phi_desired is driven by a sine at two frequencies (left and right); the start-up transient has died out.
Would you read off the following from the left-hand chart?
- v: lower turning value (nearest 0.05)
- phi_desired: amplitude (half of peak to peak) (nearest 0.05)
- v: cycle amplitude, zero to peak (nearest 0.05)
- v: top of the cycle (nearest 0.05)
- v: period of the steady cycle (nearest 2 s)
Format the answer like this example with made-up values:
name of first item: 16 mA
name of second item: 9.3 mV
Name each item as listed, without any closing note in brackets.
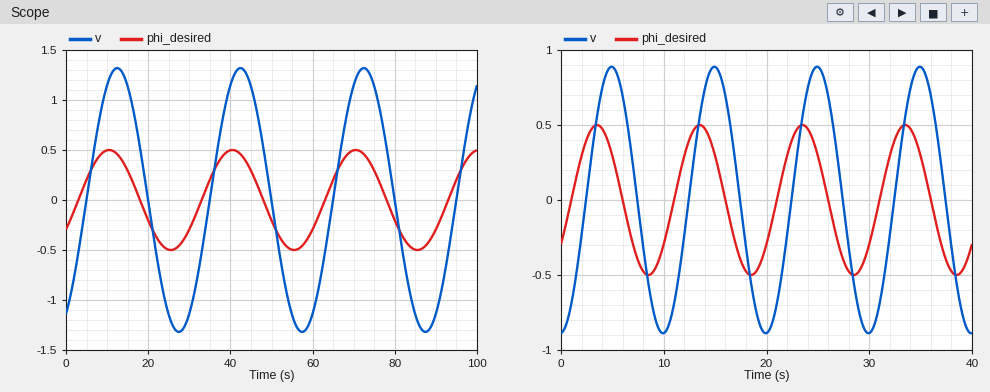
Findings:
v: lower turning value: -1.30
phi_desired: amplitude (half of peak to peak): 0.50
v: cycle amplitude, zero to peak: 1.30
v: top of the cycle: 1.30
v: period of the steady cycle: 30 s
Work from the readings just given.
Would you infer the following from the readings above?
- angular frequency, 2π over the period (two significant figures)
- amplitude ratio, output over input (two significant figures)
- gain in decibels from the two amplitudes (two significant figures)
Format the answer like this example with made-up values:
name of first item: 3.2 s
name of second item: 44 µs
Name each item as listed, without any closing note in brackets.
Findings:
angular frequency, 2π over the period: 0.21 rad/s
amplitude ratio, output over input: 2.6
gain in decibels from the two amplitudes: 8.3 dB
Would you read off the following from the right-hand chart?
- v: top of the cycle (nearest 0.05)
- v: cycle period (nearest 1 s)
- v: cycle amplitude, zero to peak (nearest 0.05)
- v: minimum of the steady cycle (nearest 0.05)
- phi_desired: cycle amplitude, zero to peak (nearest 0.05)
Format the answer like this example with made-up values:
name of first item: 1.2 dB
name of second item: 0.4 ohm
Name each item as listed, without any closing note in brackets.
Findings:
v: top of the cycle: 0.90
v: cycle period: 10 s
v: cycle amplitude, zero to peak: 0.90
v: minimum of the steady cycle: -0.90
phi_desired: cycle amplitude, zero to peak: 0.50
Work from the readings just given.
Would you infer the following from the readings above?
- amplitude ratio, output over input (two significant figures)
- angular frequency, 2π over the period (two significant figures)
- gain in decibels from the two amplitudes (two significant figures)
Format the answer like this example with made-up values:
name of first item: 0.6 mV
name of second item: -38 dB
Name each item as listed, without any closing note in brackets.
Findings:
amplitude ratio, output over input: 1.8
angular frequency, 2π over the period: 0.63 rad/s
gain in decibels from the two amplitudes: 5.1 dB
